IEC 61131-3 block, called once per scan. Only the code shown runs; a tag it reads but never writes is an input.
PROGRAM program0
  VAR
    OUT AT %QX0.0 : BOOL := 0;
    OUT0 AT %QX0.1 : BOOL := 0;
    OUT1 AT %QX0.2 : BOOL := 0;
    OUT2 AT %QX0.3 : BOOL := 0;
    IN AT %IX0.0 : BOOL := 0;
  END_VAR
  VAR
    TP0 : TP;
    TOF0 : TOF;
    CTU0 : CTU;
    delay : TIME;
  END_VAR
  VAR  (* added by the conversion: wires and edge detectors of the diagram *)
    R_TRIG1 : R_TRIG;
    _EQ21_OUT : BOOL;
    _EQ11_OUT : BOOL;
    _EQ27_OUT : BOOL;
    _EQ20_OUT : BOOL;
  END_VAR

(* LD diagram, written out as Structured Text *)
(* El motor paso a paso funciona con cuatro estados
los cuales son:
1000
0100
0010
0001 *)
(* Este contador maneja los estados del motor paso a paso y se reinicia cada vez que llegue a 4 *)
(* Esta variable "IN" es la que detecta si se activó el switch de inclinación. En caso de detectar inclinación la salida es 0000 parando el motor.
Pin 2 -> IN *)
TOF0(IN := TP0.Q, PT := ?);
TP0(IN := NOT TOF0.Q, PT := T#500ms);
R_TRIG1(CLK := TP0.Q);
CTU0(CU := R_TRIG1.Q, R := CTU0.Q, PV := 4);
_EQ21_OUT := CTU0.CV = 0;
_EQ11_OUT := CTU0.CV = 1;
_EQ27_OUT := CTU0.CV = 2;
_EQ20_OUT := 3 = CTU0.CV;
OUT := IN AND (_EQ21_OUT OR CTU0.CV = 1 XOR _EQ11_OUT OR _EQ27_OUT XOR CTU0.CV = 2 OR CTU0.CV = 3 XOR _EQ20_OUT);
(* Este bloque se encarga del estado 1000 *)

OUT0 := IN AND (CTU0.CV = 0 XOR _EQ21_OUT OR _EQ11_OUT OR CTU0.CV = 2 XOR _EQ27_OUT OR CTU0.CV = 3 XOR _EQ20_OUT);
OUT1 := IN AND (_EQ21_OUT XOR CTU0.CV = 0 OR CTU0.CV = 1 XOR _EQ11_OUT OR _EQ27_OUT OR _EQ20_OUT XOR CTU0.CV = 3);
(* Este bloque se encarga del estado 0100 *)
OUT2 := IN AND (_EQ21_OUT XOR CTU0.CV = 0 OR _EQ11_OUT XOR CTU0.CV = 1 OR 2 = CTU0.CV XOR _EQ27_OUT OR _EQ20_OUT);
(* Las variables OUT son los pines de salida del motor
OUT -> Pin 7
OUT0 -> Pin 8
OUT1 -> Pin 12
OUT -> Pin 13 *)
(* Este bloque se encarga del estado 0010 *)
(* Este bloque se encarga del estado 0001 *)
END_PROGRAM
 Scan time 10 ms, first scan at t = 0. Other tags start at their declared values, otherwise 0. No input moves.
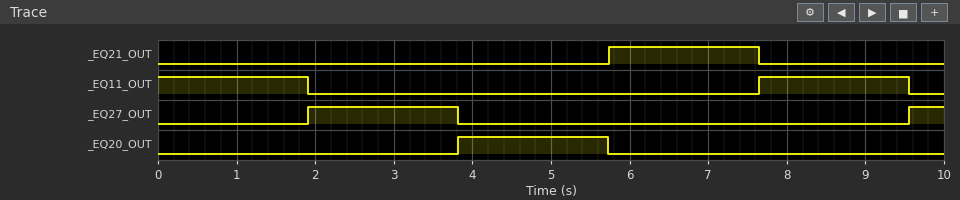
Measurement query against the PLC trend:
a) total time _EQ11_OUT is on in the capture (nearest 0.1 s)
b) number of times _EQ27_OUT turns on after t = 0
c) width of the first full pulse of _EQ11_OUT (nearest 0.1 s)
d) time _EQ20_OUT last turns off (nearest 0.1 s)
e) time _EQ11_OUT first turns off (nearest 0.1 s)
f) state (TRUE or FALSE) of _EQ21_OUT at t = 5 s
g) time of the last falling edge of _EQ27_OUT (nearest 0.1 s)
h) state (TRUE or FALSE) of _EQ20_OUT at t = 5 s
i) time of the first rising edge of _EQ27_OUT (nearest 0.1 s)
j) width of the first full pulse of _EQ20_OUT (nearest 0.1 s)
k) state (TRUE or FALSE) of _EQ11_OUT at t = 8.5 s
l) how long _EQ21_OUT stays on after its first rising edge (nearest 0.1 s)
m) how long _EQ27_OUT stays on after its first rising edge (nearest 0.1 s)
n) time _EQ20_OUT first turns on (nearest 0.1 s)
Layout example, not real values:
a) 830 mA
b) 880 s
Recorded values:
a) 3.8 s
b) 2
c) 1.9 s
d) 5.7 s
e) 1.9 s
f) FALSE
g) 3.8 s
h) TRUE
i) 1.9 s
j) 1.9 s
k) TRUE
l) 1.9 s
m) 1.9 s
n) 3.8 s
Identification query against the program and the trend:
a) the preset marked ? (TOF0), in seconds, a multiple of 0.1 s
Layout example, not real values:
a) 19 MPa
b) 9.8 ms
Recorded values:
a) 1.4 s
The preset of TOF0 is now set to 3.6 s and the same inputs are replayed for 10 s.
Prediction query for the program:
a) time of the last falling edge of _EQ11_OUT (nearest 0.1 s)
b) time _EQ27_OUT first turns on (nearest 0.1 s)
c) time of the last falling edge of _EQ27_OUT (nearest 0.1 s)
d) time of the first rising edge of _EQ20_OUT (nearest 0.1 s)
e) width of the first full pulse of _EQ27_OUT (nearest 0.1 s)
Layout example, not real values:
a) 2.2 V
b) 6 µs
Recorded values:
a) 4.1 s
b) 4.1 s
c) 8.2 s
d) 8.2 s
e) 4.1 s
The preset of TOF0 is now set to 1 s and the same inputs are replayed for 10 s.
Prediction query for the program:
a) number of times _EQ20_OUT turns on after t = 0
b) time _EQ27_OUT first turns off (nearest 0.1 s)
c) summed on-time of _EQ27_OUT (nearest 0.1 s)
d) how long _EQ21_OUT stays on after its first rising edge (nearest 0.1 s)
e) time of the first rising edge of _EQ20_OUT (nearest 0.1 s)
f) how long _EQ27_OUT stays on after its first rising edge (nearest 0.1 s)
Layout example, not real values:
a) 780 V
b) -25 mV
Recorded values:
a) 2
b) 3.0 s
c) 3.0 s
d) 1.5 s
e) 3.0 s
f) 1.5 s
